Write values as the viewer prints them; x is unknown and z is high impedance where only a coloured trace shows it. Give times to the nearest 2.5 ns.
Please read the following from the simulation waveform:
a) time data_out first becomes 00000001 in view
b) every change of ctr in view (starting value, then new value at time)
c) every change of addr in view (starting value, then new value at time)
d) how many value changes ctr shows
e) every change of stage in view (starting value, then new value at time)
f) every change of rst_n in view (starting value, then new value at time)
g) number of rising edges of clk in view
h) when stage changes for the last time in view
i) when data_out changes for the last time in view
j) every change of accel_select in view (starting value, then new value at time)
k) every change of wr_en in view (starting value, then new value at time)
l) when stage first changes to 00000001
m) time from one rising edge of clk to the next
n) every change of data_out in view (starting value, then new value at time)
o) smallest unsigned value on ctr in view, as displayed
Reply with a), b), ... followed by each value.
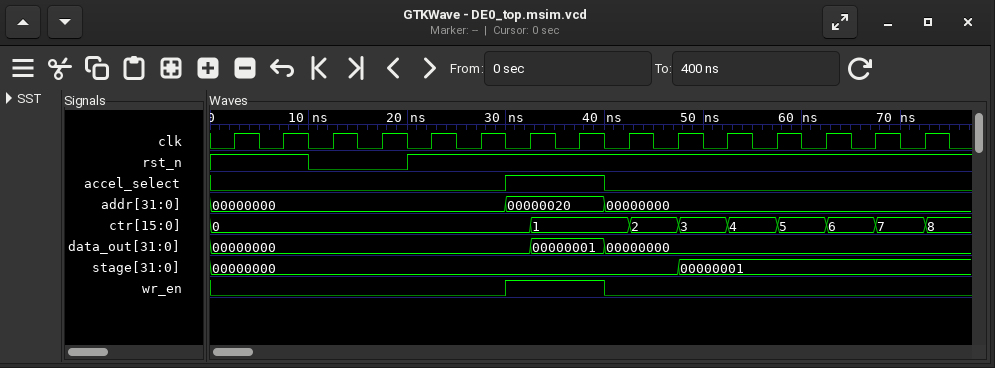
a) 32.5 ns
b) 0, 1 at 32.5 ns, 2 at 42.5 ns, 3 at 47.5 ns, 4 at 52.5 ns, 5 at 57.5 ns, 6 at 62.5 ns, 7 at 67.5 ns, 8 at 72.5 ns
c) 00000000, 00000020 at 30 ns, 00000000 at 40 ns
d) 8
e) 00000000, 00000001 at 47.5 ns
f) 1, 0 at 10 ns, 1 at 20 ns
g) 15
h) 47.5 ns
i) 40 ns
j) 0, 1 at 30 ns, 0 at 40 ns
k) 0, 1 at 30 ns, 0 at 40 ns
l) 47.5 ns
m) 5 ns
n) 00000000, 00000001 at 32.5 ns, 00000000 at 40 ns
o) 0
